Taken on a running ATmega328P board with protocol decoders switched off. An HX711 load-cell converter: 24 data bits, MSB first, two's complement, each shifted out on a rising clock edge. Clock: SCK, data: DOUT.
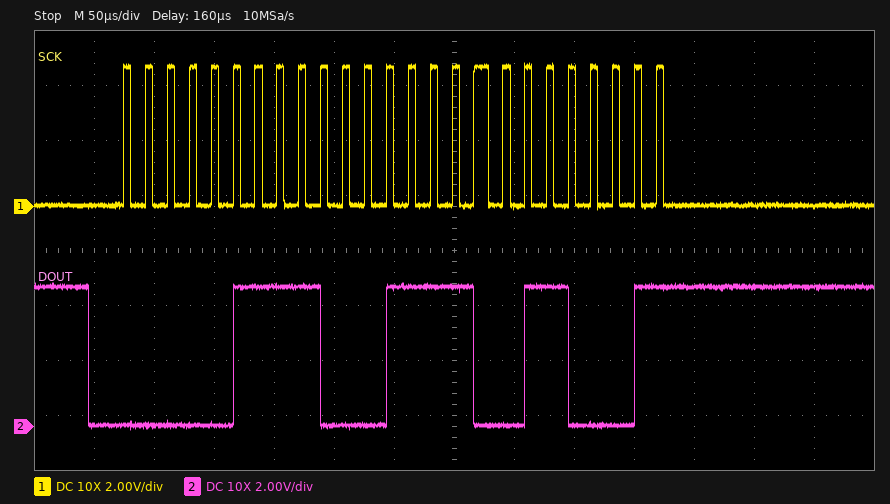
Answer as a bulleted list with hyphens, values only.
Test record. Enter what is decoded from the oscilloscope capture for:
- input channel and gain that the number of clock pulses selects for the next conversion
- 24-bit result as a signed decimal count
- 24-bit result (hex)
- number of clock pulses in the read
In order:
- channel A, gain 128
- 495409
- 0x078F31
- 25
